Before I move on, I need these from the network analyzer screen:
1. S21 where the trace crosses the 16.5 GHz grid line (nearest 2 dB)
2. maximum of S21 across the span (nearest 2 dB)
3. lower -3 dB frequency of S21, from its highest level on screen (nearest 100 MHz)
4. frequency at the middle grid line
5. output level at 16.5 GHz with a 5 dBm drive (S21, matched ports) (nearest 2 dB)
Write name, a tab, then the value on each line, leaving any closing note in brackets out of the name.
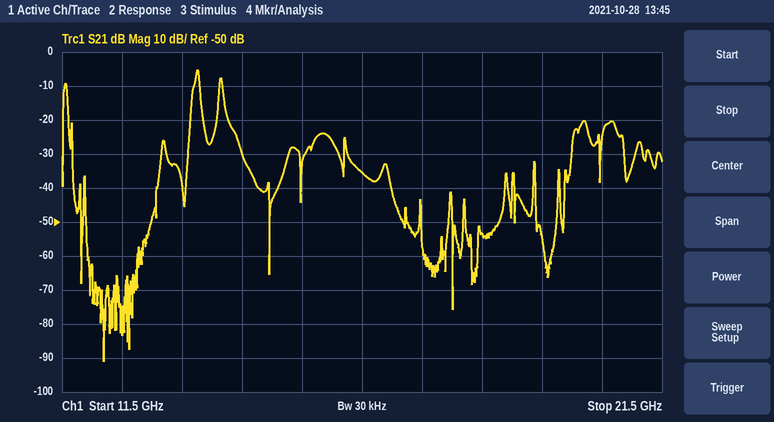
S21 where the trace crosses the 16.5 GHz grid line	-36 dB
maximum of S21 across the span	-6 dB
lower -3 dB frequency of S21, from its highest level on screen	13.7 GHz
frequency at the middle grid line	16.5 GHz
output level at 16.5 GHz with a 5 dBm drive (S21, matched ports)	-30 dBm
